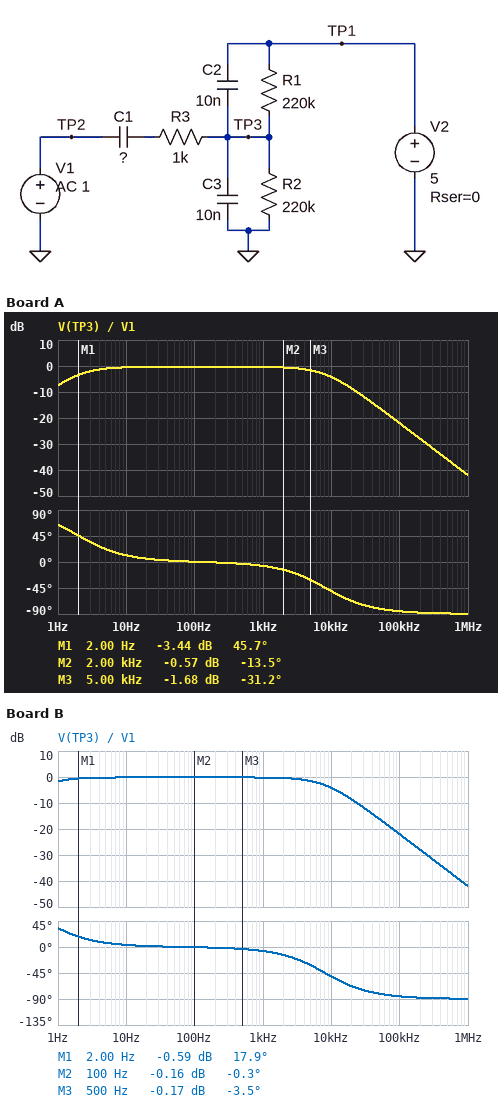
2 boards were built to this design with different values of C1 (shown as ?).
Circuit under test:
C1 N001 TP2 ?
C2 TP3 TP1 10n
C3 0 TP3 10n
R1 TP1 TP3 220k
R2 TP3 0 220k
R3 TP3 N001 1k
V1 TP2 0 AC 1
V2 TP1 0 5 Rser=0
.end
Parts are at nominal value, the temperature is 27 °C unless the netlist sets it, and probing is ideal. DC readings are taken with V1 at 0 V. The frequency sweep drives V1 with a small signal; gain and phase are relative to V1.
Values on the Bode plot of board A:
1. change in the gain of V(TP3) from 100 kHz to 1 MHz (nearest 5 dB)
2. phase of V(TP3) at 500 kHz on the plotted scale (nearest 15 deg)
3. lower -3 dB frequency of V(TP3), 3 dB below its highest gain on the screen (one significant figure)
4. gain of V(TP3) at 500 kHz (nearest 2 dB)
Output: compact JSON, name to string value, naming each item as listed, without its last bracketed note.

{"change in the gain of V(TP3) from 100 kHz to 1 MHz": "-20 dB", "phase of V(TP3) at 500 kHz on the plotted scale": "-90 deg", "lower -3 dB frequency of V(TP3), 3 dB below its highest gain on the screen": "2 Hz", "gain of V(TP3) at 500 kHz": "-36 dB"}
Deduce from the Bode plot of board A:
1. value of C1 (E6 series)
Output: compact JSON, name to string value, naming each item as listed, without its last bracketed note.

{"value of C1": "680 nF"}
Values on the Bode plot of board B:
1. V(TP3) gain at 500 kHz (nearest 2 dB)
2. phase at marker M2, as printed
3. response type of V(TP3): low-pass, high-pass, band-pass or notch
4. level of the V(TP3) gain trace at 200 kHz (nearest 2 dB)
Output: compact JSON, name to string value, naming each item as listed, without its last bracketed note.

{"V(TP3) gain at 500 kHz": "-36 dB", "phase at marker M2, as printed": "-0.3 deg", "response type of V(TP3): low-pass, high-pass, band-pass or notch": "low-pass", "level of the V(TP3) gain trace at 200 kHz": "-28 dB"}
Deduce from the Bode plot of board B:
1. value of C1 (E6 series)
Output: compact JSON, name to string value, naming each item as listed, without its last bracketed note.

{"value of C1": "2.2 µF"}
